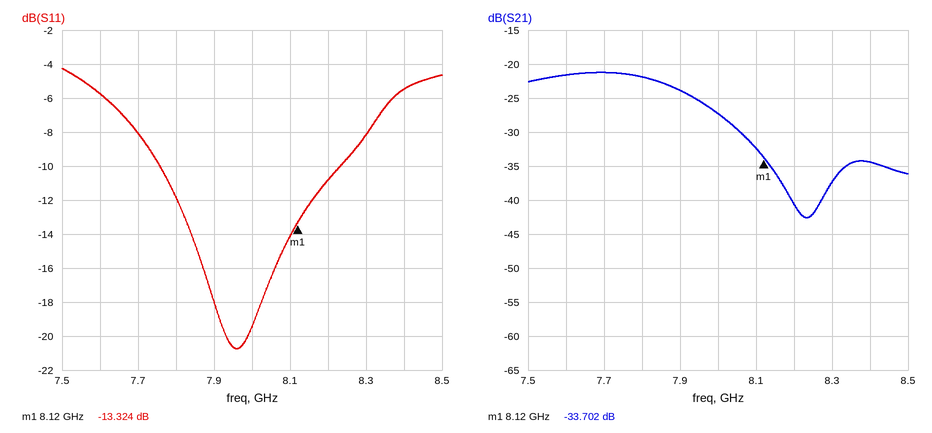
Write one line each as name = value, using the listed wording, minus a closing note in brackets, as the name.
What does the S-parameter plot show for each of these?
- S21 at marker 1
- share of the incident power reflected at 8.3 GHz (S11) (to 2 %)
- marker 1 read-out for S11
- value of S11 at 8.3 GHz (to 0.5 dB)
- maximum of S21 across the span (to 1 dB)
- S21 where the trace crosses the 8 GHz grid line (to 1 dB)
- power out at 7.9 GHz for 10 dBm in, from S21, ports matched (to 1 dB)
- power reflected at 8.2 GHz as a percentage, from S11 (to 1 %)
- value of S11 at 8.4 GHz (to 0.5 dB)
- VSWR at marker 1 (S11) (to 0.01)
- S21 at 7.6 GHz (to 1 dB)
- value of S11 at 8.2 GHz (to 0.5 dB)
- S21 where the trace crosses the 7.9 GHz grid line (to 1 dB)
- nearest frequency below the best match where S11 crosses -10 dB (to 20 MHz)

S21 at marker 1 = -33.702 dB
share of the incident power reflected at 8.3 GHz (S11) = 16 %
marker 1 read-out for S11 = -13.324 dB
value of S11 at 8.3 GHz = -8.0 dB
maximum of S21 across the span = -21 dB
S21 where the trace crosses the 8 GHz grid line = -27 dB
power out at 7.9 GHz for 10 dBm in, from S21, ports matched = -14 dBm
power reflected at 8.2 GHz as a percentage, from S11 = 8 %
value of S11 at 8.4 GHz = -5.5 dB
VSWR at marker 1 (S11) = 1.55
S21 at 7.6 GHz = -22 dB
value of S11 at 8.2 GHz = -11.0 dB
S21 where the trace crosses the 7.9 GHz grid line = -24 dB
nearest frequency below the best match where S11 crosses -10 dB = 7.76 GHz
